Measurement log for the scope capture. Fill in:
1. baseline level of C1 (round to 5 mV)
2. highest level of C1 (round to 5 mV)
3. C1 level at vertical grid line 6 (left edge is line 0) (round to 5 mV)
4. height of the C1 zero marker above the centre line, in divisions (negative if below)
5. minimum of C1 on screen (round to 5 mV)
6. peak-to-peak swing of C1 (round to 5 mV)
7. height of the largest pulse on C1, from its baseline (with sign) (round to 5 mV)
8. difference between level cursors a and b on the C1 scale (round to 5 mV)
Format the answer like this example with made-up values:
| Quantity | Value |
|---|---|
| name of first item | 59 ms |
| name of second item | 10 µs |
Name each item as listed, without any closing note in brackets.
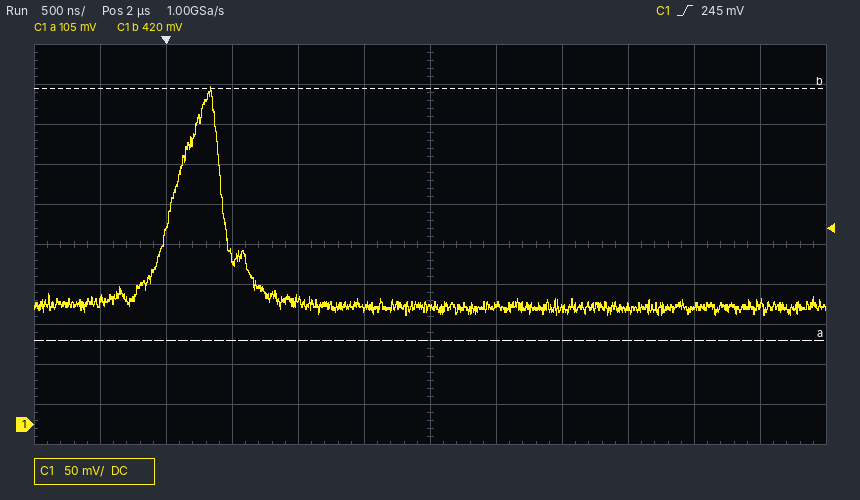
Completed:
| Quantity | Value |
|---|---|
| baseline level of C1 | 145 mV |
| highest level of C1 | 420 mV |
| C1 level at vertical grid line 6 (left edge is line 0) | 145 mV |
| height of the C1 zero marker above the centre line, in divisions | -4.5 div |
| minimum of C1 on screen | 135 mV |
| peak-to-peak swing of C1 | 285 mV |
| height of the largest pulse on C1, from its baseline (with sign) | +275 mV |
| difference between level cursors a and b on the C1 scale | 315 mV |
